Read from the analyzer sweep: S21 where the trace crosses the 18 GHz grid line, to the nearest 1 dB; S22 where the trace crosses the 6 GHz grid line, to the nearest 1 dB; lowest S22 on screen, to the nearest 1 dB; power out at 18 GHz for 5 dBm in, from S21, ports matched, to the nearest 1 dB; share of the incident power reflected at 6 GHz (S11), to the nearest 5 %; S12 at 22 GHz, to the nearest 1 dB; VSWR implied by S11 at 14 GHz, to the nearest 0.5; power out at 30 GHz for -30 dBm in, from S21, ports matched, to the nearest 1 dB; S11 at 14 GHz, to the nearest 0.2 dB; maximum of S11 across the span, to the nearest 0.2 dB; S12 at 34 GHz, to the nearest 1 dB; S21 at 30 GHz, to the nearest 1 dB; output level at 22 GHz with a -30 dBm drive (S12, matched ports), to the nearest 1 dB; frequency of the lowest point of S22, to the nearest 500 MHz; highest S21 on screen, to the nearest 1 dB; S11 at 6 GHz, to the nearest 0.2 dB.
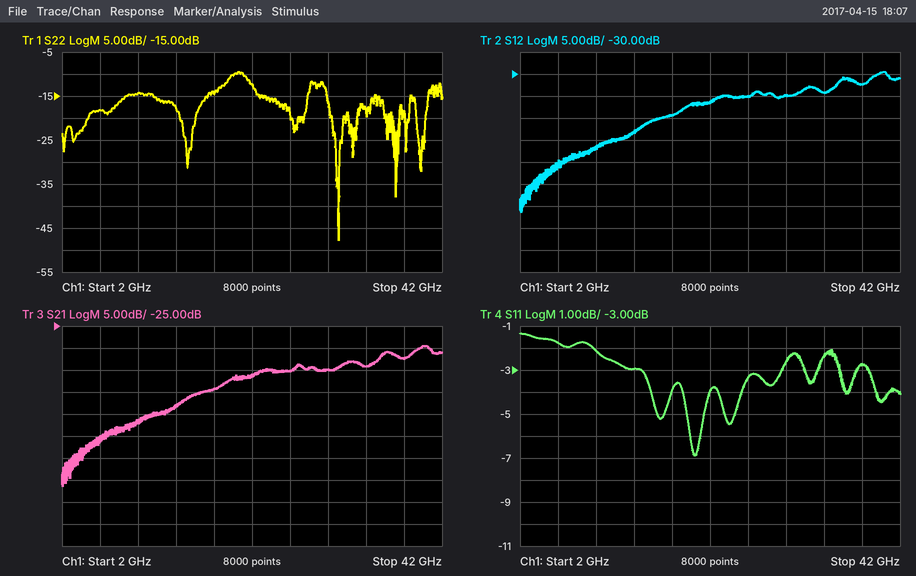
-39 dB
-18 dB
-48 dB
-34 dBm
65 %
-36 dB
6.0
-65 dBm
-3.0 dB
-1.4 dB
-34 dB
-35 dB
-66 dBm
31.0 GHz
-29 dB
-1.8 dB
